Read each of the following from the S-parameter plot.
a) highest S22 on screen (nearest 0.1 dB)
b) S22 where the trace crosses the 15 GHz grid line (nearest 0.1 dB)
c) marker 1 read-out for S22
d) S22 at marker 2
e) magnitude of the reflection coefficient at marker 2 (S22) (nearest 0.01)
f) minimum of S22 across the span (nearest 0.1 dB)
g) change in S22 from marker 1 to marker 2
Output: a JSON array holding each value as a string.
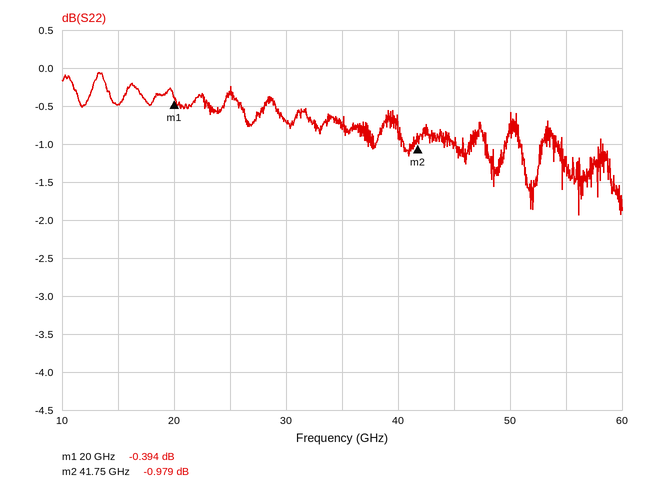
["-0.1 dB", "-0.5 dB", "-0.394 dB", "-0.979 dB", "0.89", "-1.9 dB", "-0.585 dB"]
